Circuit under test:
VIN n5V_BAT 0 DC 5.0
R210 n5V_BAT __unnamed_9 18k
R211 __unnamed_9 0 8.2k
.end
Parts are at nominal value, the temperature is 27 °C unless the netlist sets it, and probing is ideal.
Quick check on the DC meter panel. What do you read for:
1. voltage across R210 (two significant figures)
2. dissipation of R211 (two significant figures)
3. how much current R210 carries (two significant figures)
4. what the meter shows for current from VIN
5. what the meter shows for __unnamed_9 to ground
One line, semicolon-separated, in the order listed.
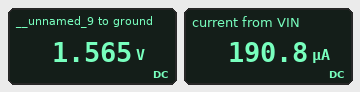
3.4 V; 300 µW; 190 µA; 190.8 µA; 1.565 V
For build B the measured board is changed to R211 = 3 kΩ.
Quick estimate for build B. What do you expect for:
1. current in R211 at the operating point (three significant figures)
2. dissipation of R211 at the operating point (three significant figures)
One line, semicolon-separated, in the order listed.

238 µA; 170 µW
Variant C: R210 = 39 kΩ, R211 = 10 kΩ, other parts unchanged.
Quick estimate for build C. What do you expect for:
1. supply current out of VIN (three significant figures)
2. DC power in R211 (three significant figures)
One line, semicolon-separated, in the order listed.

102 µA; 104 µW
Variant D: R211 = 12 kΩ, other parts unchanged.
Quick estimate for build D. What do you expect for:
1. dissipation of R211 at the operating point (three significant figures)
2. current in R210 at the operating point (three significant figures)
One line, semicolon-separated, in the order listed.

333 µW; 167 µA
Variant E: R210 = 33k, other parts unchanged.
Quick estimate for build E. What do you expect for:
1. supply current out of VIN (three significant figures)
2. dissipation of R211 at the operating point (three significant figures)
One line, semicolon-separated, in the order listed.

121 µA; 121 µW
